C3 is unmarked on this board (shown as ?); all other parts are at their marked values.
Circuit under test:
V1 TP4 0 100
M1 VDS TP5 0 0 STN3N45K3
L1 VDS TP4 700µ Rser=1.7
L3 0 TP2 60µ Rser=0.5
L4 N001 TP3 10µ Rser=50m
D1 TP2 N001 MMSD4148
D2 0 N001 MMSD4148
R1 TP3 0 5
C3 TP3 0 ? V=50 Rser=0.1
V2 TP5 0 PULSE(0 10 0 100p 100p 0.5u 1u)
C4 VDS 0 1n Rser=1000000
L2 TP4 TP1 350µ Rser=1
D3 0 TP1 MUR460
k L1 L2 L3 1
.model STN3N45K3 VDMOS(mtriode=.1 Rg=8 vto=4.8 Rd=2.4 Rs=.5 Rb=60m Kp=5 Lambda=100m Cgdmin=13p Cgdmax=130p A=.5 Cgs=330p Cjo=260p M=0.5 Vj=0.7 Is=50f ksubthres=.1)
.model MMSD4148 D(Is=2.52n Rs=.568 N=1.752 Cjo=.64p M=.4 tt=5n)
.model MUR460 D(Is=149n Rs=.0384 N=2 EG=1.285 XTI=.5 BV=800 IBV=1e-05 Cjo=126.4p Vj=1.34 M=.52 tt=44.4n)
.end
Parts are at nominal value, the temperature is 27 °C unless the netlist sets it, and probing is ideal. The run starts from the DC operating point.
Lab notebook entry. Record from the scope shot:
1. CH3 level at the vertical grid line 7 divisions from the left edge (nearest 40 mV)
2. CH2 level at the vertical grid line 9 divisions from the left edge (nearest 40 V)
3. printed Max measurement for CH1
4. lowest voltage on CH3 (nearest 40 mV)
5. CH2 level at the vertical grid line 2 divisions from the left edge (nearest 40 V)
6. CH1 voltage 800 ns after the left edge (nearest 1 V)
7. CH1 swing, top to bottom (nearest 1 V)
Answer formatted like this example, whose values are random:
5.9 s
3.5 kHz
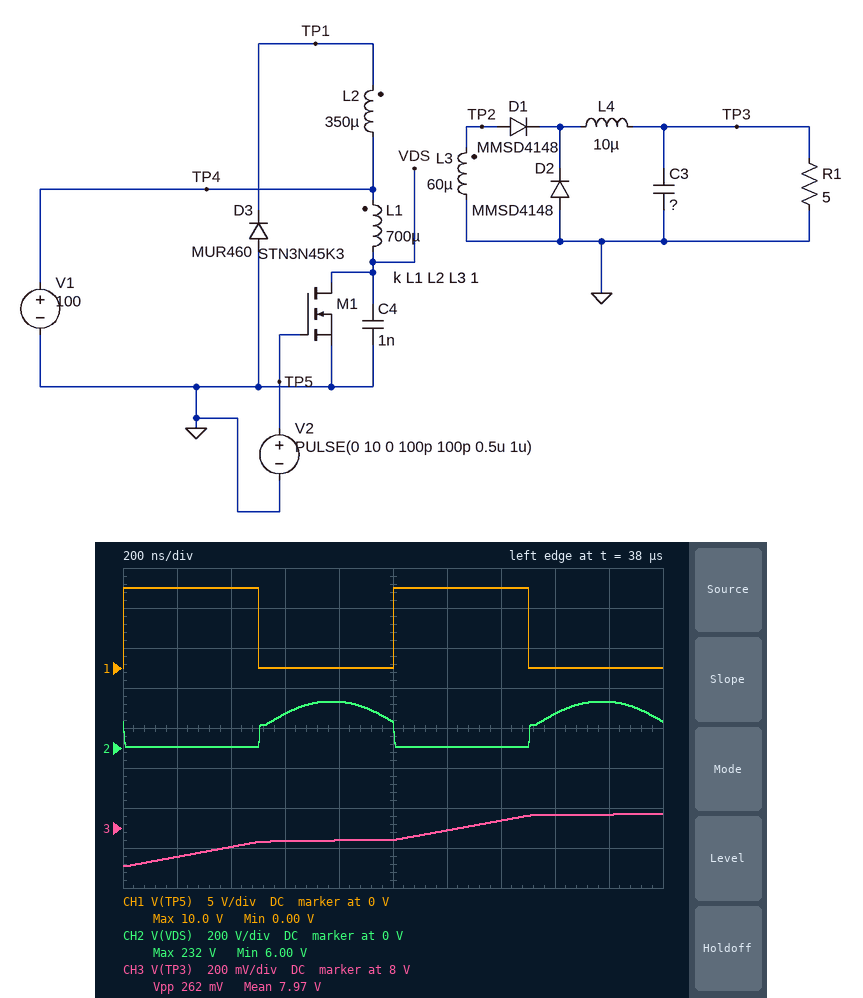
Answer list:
8.04 V
240 V
10.0 V
7.80 V
0 V
0 V
10 V
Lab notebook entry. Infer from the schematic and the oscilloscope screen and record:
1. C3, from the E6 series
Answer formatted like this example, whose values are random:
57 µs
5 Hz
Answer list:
33 µF
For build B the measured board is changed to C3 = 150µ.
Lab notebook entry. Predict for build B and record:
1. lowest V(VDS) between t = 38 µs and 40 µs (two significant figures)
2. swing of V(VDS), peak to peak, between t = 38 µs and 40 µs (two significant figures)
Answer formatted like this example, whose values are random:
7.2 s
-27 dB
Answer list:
9.6 V
220 V
